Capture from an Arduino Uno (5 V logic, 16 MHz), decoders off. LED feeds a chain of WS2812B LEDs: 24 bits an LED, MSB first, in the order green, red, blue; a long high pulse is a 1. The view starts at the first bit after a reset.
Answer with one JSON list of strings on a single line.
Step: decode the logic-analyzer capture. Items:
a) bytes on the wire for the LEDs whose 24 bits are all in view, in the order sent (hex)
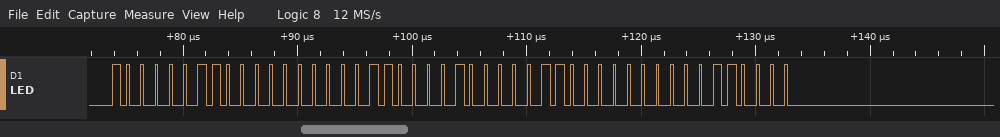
["83 00 30 83 00 30"]
